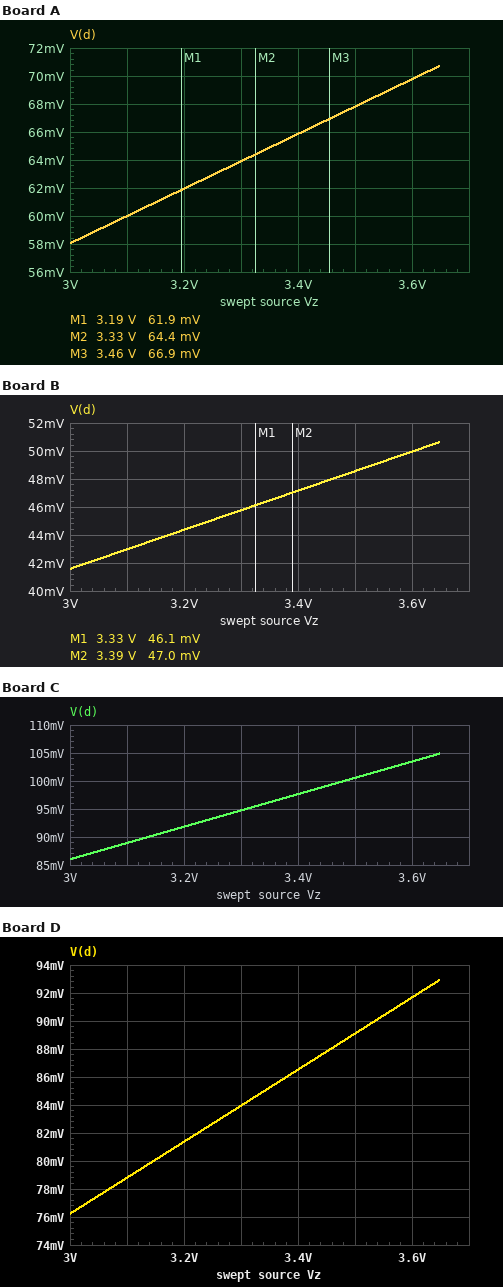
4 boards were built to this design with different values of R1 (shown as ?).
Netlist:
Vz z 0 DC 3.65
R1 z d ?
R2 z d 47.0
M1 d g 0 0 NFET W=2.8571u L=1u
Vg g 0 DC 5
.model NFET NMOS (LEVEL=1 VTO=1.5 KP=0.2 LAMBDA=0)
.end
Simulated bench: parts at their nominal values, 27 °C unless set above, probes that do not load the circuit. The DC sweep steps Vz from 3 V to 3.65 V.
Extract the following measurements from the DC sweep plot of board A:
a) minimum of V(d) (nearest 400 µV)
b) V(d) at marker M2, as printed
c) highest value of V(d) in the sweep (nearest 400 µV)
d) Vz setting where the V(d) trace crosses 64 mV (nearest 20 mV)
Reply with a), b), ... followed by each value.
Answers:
a) 58.0 mV
b) 64.4 mV
c) 70.8 mV
d) 3.30 V
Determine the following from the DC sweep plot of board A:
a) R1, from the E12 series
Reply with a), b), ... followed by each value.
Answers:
a) 56 Ω
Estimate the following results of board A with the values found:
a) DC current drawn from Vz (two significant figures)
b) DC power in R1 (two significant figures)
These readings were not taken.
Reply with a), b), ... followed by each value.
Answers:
a) 140 mA
b) 230 mW
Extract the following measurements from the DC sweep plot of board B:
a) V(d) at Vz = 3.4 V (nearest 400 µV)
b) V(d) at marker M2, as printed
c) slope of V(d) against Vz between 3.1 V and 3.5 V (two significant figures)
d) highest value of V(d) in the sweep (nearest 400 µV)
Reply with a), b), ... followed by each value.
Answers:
a) 47.2 mV
b) 47.0 mV
c) 0.014 V/V
d) 50.8 mV
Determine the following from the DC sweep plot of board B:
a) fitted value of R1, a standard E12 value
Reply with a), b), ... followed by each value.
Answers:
a) 150 Ω
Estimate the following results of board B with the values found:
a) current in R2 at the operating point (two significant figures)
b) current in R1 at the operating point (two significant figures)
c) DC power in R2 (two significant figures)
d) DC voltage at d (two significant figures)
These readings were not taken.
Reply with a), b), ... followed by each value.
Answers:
a) 77 mA
b) 24 mA
c) 280 mW
d) 51 mV
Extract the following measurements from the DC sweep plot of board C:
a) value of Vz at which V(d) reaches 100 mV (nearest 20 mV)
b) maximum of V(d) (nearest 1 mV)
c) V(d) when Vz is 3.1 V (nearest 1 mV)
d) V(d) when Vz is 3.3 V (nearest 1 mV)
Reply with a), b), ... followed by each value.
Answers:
a) 3.48 V
b) 105 mV
c) 89 mV
d) 95 mV
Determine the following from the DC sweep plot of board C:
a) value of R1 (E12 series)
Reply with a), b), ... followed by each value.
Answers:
a) 27 Ω
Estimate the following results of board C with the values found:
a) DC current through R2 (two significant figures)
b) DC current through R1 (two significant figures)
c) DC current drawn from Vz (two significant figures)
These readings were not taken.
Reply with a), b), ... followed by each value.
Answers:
a) 75 mA
b) 130 mA
c) 210 mA
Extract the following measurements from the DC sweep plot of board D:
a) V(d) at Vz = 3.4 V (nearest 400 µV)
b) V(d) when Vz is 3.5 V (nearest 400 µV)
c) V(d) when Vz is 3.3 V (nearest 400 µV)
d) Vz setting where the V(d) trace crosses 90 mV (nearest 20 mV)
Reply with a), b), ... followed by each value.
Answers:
a) 86.4 mV
b) 89.2 mV
c) 84.0 mV
d) 3.54 V
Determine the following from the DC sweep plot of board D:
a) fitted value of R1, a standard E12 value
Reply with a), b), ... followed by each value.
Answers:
a) 33 Ω
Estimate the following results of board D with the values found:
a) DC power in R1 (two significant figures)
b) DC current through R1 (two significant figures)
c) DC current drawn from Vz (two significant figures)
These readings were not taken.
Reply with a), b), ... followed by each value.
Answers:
a) 380 mW
b) 110 mA
c) 180 mA
